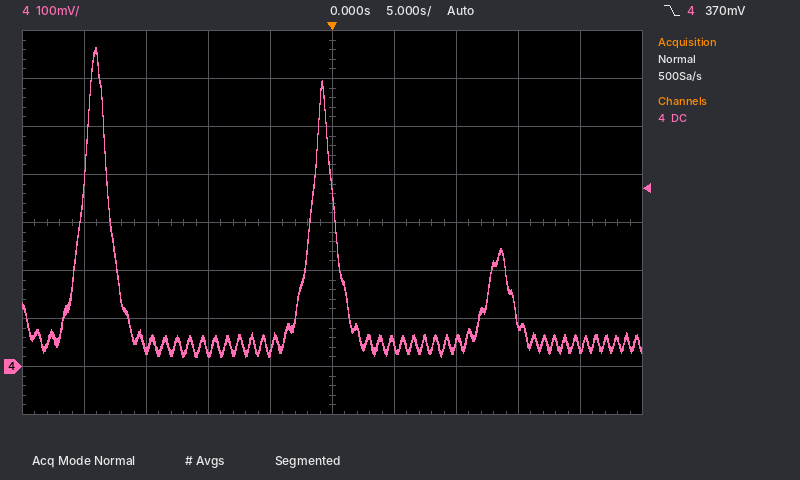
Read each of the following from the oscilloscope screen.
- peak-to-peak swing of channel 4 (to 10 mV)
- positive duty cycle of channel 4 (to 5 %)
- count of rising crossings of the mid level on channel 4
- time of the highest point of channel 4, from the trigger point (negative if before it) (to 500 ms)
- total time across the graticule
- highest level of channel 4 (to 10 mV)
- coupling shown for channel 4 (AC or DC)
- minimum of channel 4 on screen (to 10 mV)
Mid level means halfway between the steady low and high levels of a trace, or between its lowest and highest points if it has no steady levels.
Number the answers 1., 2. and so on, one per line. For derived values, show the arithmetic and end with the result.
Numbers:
1. 660 mV − (20 mV) = 640 mV
2. 10 %
3. 2
4. -19.0 s
5. 50 s
6. 660 mV
7. DC
8. 20 mV
